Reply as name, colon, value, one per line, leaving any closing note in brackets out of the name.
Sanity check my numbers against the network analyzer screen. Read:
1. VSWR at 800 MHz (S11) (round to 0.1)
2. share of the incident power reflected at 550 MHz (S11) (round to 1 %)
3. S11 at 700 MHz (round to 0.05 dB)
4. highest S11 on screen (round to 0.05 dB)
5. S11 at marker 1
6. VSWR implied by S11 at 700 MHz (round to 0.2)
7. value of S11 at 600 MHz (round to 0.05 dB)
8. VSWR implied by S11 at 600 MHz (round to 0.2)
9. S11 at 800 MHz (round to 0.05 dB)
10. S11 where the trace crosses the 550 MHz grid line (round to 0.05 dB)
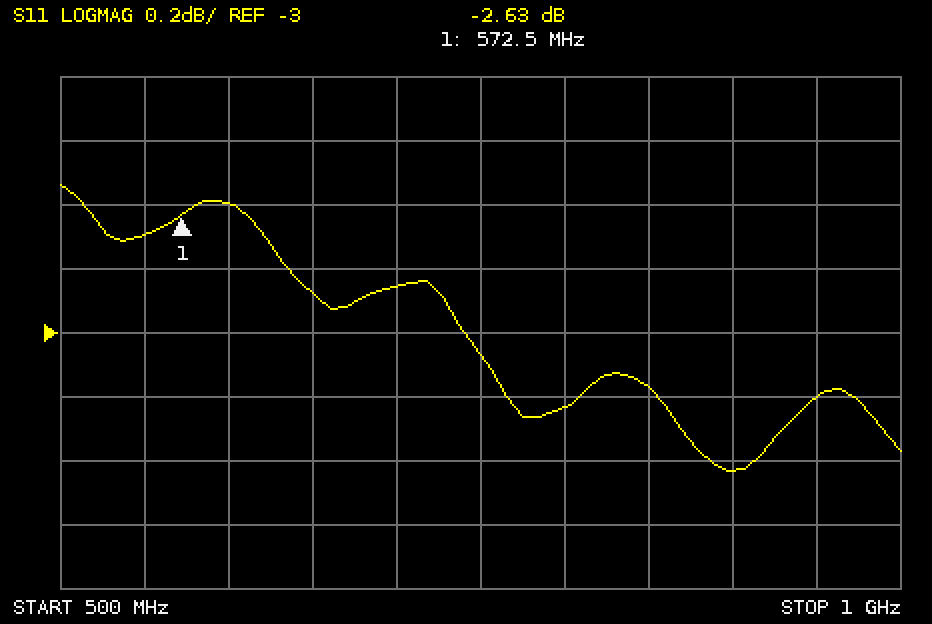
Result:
VSWR at 800 MHz (S11): 5.4
share of the incident power reflected at 550 MHz (S11): 54 %
S11 at 700 MHz: -2.85 dB
highest S11 on screen: -2.55 dB
S11 at marker 1: -2.63 dB
VSWR implied by S11 at 700 MHz: 6.2
value of S11 at 600 MHz: -2.60 dB
VSWR implied by S11 at 600 MHz: 6.8
S11 at 800 MHz: -3.25 dB
S11 where the trace crosses the 550 MHz grid line: -2.70 dB
